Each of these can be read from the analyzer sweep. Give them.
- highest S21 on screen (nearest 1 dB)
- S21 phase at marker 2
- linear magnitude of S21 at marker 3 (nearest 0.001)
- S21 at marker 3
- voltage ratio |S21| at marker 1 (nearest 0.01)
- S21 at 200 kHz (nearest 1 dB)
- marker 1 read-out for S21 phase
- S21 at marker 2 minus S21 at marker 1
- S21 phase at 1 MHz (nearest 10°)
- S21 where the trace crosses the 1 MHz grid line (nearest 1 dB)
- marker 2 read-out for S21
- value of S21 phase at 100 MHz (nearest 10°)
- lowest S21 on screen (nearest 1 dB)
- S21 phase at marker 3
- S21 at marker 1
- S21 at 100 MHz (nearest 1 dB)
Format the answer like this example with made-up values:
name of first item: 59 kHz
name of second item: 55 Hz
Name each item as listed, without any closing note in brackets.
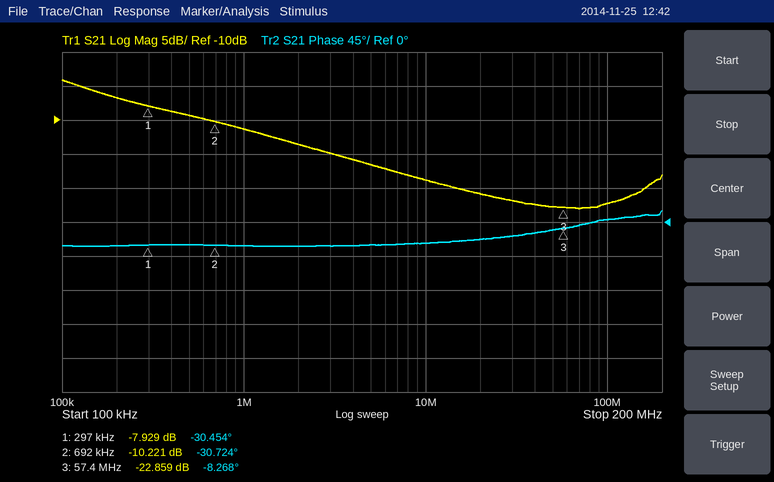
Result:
highest S21 on screen: -4 dB
S21 phase at marker 2: -30.724°
linear magnitude of S21 at marker 3: 0.072
S21 at marker 3: -22.859 dB
voltage ratio |S21| at marker 1: 0.40
S21 at 200 kHz: -7 dB
marker 1 read-out for S21 phase: -30.454°
S21 at marker 2 minus S21 at marker 1: -2.292 dB
S21 phase at 1 MHz: -30°
S21 where the trace crosses the 1 MHz grid line: -11 dB
marker 2 read-out for S21: -10.221 dB
value of S21 phase at 100 MHz: 0°
lowest S21 on screen: -23 dB
S21 phase at marker 3: -8.268°
S21 at marker 1: -7.929 dB
S21 at 100 MHz: -22 dB
